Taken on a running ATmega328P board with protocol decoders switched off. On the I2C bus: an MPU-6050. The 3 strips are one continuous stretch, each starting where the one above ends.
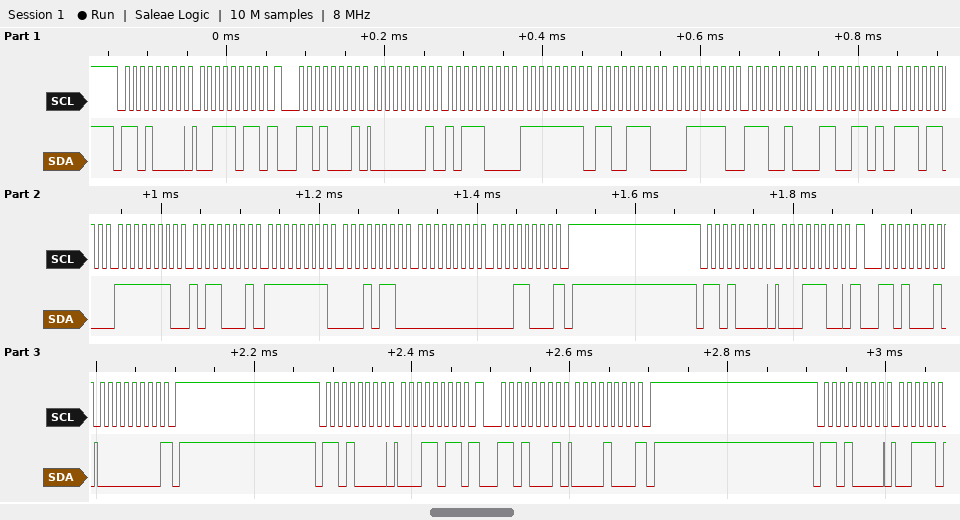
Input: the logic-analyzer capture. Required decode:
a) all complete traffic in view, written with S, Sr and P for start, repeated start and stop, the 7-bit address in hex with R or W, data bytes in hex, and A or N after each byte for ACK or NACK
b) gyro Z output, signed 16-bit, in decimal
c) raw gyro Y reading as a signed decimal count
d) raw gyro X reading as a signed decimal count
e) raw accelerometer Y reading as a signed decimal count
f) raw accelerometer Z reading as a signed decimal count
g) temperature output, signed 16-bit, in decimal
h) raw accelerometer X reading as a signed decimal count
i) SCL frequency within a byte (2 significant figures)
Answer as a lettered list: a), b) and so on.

a) S 68W A 3B A Sr 68R A 01 A B8 A FF A CE A 3E A E4 A CD A EC A FE A B1 A FF A 16 A 00 A 18 N P S 68W A 1C A Sr 68R A 00 N P S 68W A 1B A Sr 68R A 08 N P S 68W A
b) 24
c) -234
d) -335
e) -50
f) 16100
g) -12820
h) 440
i) 100 kHz
